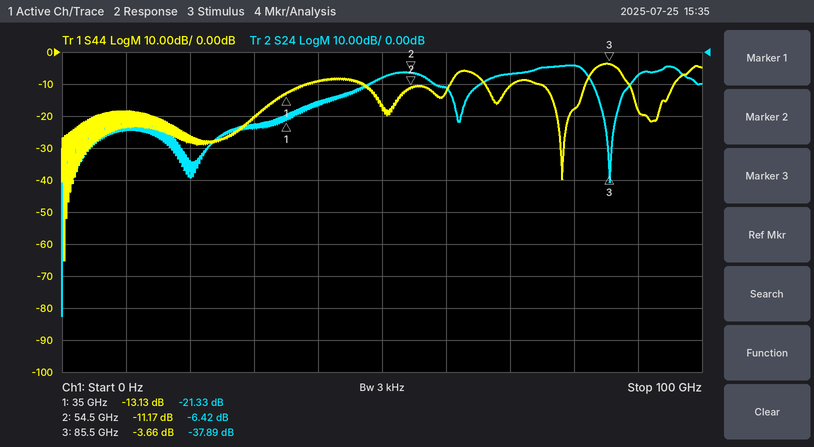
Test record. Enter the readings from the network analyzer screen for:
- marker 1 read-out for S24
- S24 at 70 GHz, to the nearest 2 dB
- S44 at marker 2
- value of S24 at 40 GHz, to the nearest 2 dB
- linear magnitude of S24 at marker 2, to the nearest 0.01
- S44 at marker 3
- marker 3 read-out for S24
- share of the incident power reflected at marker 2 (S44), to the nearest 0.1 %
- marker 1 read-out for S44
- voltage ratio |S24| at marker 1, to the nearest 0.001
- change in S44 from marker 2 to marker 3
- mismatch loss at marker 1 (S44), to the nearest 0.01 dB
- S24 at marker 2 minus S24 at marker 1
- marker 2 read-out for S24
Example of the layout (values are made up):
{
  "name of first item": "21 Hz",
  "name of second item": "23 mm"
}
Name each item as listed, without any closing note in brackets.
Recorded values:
{
  "marker 1 read-out for S24": "-21.33 dB",
  "S24 at 70 GHz, to the nearest 2 dB": "-6 dB",
  "S44 at marker 2": "-11.17 dB",
  "value of S24 at 40 GHz, to the nearest 2 dB": "-16 dB",
  "linear magnitude of S24 at marker 2, to the nearest 0.01": "0.48",
  "S44 at marker 3": "-3.66 dB",
  "marker 3 read-out for S24": "-37.89 dB",
  "share of the incident power reflected at marker 2 (S44), to the nearest 0.1 %": "7.6 %",
  "marker 1 read-out for S44": "-13.13 dB",
  "voltage ratio |S24| at marker 1, to the nearest 0.001": "0.086",
  "change in S44 from marker 2 to marker 3": "7.51 dB",
  "mismatch loss at marker 1 (S44), to the nearest 0.01 dB": "0.22 dB",
  "S24 at marker 2 minus S24 at marker 1": "14.91 dB",
  "marker 2 read-out for S24": "-6.42 dB"
}
